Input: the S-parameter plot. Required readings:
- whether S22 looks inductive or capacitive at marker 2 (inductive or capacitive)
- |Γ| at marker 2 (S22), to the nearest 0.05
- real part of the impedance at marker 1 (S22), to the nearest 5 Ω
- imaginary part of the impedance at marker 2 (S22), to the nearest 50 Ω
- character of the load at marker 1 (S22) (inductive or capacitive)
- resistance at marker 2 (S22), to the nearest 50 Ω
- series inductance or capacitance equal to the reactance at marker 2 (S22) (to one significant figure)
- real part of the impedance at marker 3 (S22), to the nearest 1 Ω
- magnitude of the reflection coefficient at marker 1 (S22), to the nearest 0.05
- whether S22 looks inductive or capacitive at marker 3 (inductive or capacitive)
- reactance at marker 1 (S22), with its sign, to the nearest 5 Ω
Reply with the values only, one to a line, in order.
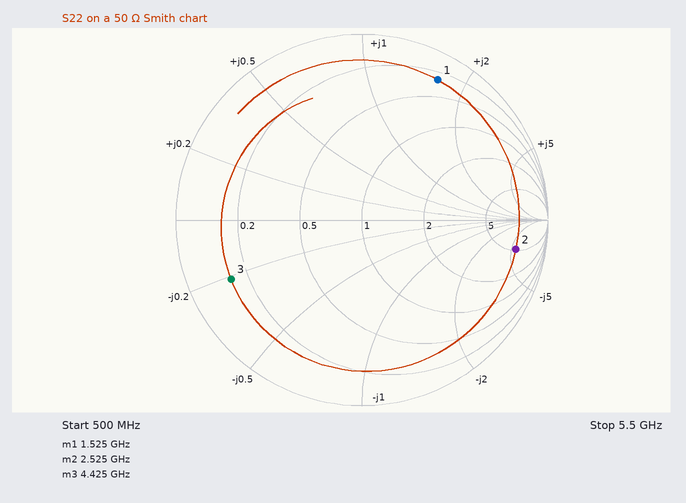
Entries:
capacitive
0.85
15 Ω
-300 Ω
inductive
250 Ω
200 fF
7 Ω
0.85
capacitive
+80 Ω
